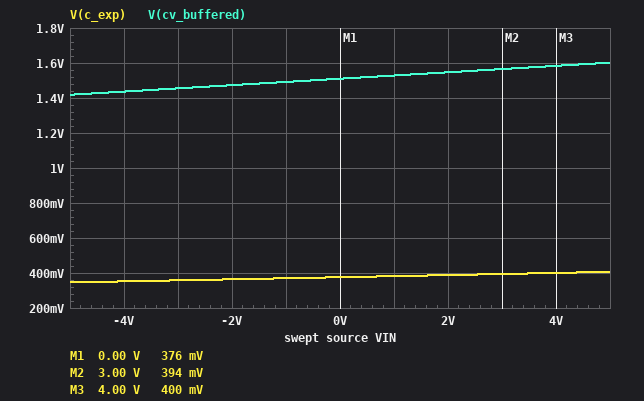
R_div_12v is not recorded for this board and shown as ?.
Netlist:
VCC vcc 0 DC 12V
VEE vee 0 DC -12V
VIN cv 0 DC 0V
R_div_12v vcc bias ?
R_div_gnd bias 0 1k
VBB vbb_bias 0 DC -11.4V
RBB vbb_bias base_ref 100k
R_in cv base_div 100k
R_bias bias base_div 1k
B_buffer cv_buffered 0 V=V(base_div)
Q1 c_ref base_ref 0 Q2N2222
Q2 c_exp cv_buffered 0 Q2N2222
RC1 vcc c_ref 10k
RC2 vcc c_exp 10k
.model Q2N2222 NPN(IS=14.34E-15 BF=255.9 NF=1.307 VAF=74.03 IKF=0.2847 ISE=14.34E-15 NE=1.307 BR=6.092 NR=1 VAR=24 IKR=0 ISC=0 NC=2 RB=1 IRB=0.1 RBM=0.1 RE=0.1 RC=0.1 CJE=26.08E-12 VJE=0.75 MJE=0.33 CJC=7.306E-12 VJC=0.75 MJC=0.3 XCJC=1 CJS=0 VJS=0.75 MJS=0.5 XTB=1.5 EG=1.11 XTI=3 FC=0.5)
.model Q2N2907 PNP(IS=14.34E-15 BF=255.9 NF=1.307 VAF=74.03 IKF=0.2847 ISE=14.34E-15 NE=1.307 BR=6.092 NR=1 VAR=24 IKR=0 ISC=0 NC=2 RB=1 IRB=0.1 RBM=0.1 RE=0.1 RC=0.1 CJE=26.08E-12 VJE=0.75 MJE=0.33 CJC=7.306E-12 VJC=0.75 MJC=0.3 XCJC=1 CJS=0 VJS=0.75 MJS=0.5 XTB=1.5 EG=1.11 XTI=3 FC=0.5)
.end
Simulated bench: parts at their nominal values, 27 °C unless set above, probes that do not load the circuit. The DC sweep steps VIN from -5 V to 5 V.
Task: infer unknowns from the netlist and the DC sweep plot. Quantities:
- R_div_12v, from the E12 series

6.8 kΩ
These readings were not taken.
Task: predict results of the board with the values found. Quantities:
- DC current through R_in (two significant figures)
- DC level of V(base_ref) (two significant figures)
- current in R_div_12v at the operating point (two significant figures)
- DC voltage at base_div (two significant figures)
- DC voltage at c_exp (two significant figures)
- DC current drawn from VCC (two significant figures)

15 µA
-11 V
1.5 mA
1.5 V
380 mV
2.7 mA
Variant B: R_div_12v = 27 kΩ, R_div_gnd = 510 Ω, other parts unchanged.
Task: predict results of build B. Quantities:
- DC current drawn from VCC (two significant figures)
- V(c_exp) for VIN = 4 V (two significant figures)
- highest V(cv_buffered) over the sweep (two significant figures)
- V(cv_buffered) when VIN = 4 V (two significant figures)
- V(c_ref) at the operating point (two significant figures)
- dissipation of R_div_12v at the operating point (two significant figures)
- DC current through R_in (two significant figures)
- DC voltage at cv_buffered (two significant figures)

440 µA
12 V
290 mV
280 mV
12 V
5.1 mW
2.2 µA
220 mV
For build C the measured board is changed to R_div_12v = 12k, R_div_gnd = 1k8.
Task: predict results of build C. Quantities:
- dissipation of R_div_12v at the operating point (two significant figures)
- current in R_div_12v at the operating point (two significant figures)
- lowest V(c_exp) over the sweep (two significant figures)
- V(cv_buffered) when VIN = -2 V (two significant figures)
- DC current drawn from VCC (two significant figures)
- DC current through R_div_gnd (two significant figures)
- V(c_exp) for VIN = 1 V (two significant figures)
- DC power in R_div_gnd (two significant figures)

9.1 mW
870 µA
340 mV
1.5 V
2.0 mA
860 µA
390 mV
1.3 mW
